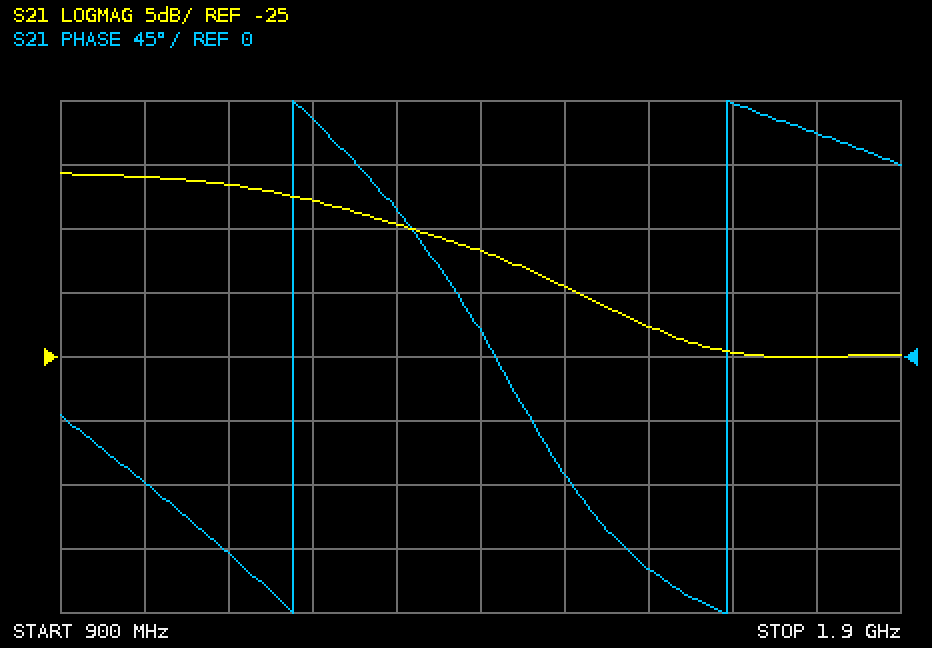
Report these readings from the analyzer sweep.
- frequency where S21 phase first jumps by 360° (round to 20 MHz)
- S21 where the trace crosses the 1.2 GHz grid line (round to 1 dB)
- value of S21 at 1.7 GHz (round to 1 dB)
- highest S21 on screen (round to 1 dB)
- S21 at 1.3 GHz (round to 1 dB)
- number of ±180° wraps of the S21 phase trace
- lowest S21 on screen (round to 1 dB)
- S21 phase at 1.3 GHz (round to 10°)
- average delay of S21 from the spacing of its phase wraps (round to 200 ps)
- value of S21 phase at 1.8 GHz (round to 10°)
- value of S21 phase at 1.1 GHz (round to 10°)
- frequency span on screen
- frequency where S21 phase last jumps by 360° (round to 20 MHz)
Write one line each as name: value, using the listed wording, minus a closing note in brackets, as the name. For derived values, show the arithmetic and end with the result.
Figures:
frequency where S21 phase first jumps by 360°: 1.18 GHz
S21 where the trace crosses the 1.2 GHz grid line: -13 dB
value of S21 at 1.7 GHz: -25 dB
highest S21 on screen: -11 dB
S21 at 1.3 GHz: -15 dB
number of ±180° wraps of the S21 phase trace: 2
lowest S21 on screen: -25 dB
S21 phase at 1.3 GHz: 100°
average delay of S21 from the spacing of its phase wraps: 1 cycle / (1.70 GHz − 1.18 GHz) ≈ 1.92 ns, so 2.0 ns to the nearest 200 ps
value of S21 phase at 1.8 GHz: 160°
value of S21 phase at 1.1 GHz: -140°
frequency span on screen: 1 GHz
frequency where S21 phase last jumps by 360°: 1.70 GHz
